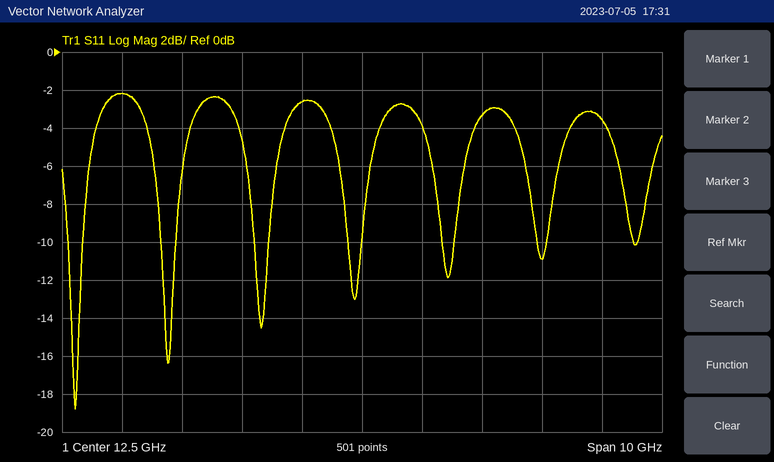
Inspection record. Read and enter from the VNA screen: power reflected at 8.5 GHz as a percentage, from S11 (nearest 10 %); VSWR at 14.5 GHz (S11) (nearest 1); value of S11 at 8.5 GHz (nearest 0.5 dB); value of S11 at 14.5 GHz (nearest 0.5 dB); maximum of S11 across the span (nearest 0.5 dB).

60 %
5
-2.0 dB
-3.5 dB
-2.0 dB
